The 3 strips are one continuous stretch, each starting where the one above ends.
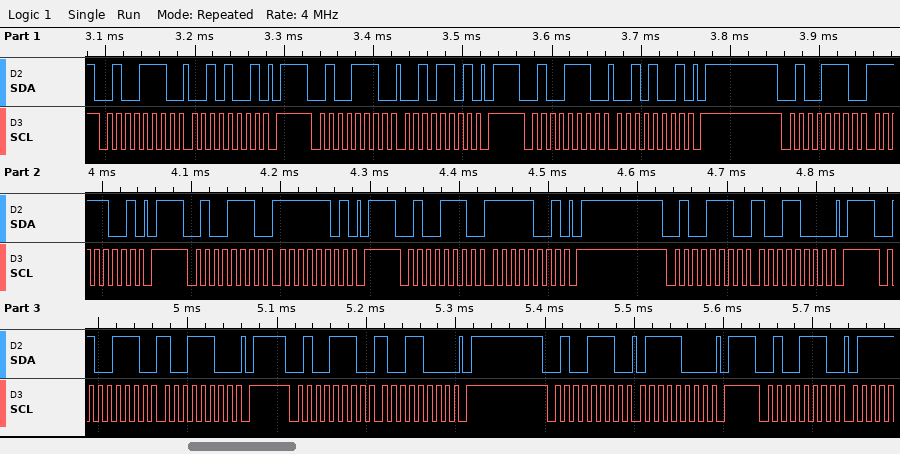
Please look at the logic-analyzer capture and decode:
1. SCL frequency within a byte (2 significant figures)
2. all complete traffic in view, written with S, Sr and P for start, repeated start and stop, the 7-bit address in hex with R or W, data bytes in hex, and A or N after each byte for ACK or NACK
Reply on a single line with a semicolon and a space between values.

100 kHz; S 27W A 29 A P S 27W A 2D A P S 27W A 29 A P S 27W A F9 A P S 27W A FD A P S 27W A F9 A P S 27W A 98 A P S 27W A 9C A P S 27W A 98 A P S 27W A 78 A P S 27W A
